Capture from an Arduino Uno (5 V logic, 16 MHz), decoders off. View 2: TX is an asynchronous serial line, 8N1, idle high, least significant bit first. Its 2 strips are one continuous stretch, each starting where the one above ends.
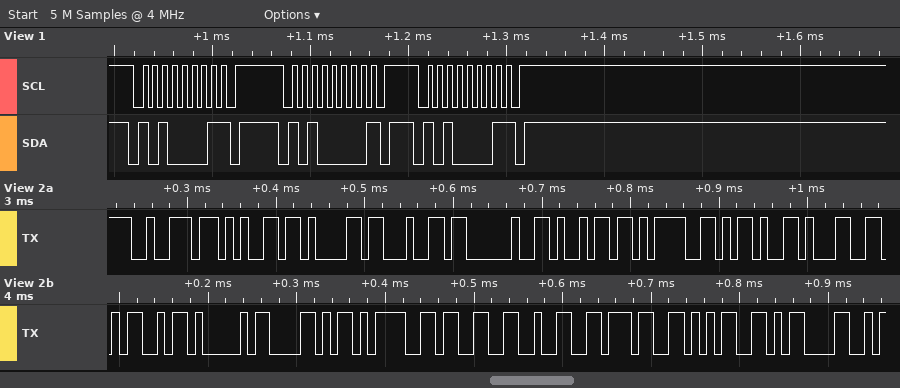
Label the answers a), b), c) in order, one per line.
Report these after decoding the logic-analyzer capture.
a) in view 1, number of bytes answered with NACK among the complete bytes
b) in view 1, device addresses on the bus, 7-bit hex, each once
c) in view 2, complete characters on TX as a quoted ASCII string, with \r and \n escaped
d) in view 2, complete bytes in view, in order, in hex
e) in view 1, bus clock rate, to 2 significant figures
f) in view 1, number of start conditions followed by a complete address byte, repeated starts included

a) 3
b) 0x50
c) "read i=-1MAX=3275\r"
d) 72 65 61 64 20 69 3D 2D 31 4D 41 58 3D 33 32 37 35 0D
e) 100 kHz
f) 3
